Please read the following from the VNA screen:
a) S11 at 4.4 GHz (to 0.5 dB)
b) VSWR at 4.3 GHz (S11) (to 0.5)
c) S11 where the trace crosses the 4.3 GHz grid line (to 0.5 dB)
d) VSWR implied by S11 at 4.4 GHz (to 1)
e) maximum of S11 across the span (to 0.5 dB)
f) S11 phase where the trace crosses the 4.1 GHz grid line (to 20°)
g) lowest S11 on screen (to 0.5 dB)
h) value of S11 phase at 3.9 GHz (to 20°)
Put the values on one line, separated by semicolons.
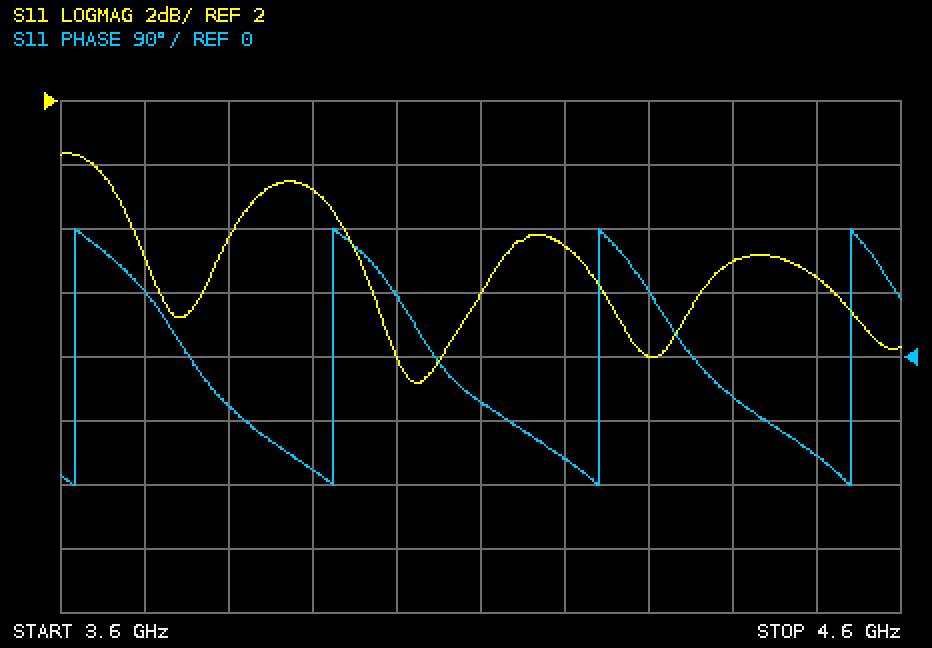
-3.0 dB; 3.0; -6.0 dB; 6; 0.5 dB; -60°; -7.0 dB; -160°
